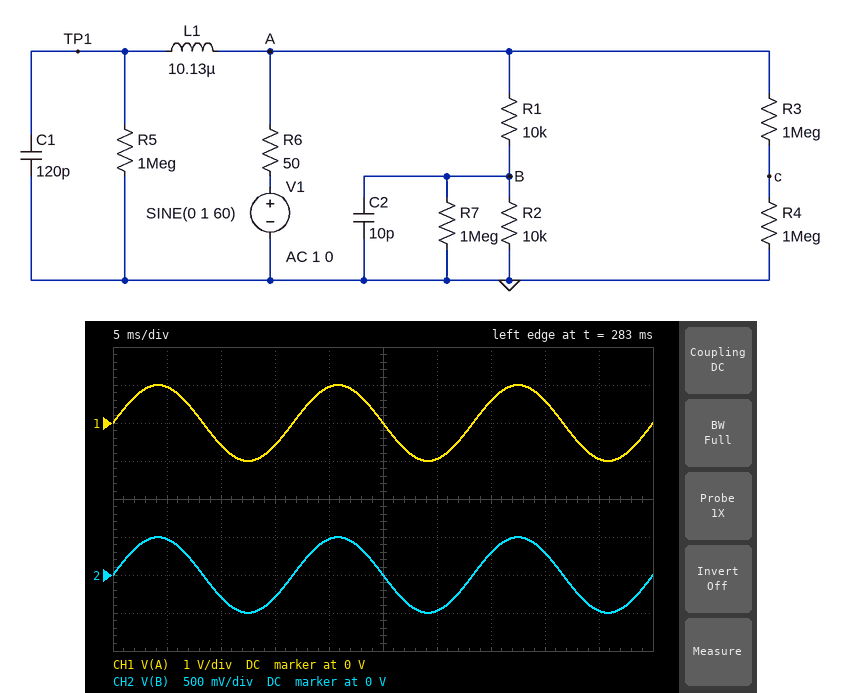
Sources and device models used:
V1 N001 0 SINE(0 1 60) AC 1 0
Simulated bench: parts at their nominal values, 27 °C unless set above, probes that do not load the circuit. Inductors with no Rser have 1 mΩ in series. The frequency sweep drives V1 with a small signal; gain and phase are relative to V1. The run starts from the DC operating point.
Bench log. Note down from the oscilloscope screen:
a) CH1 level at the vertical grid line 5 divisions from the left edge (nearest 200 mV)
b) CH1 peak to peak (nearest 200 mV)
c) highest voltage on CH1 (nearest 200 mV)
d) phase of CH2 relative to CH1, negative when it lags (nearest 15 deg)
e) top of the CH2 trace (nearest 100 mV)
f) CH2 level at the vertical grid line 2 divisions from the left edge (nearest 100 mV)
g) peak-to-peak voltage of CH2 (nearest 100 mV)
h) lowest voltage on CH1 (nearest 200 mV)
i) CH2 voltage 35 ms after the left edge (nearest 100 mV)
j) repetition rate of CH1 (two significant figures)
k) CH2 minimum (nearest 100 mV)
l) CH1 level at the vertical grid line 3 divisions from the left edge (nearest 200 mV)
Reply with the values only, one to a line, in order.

0 V
2.0 V
1.0 V
0 deg
500 mV
-300 mV
1.0 V
-1.0 V
300 mV
60 Hz
-500 mV
-600 mV
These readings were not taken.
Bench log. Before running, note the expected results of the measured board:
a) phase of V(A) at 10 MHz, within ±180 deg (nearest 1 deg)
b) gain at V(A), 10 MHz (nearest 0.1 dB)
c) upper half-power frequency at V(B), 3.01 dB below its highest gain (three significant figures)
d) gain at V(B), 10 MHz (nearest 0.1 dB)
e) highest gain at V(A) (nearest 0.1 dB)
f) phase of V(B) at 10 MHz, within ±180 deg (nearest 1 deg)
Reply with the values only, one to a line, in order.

6 deg
-0.1 dB
3.05 MHz
-16.5 dB
0 dB
-67 deg
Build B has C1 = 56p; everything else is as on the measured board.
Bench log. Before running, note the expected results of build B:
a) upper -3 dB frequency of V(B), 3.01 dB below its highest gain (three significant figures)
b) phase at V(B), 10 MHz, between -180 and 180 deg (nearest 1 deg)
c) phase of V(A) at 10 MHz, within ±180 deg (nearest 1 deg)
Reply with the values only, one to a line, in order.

3.17 MHz
-64 deg
8 deg
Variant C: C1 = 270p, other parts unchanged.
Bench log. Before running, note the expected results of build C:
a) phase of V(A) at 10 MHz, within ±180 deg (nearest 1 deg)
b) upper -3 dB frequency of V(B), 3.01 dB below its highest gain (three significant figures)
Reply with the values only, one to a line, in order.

5 deg
2.39 MHz
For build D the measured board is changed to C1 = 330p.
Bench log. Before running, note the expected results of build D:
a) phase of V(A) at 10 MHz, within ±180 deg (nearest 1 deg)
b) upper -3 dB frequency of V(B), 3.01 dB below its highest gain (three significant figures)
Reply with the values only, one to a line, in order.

5 deg
2.18 MHz
